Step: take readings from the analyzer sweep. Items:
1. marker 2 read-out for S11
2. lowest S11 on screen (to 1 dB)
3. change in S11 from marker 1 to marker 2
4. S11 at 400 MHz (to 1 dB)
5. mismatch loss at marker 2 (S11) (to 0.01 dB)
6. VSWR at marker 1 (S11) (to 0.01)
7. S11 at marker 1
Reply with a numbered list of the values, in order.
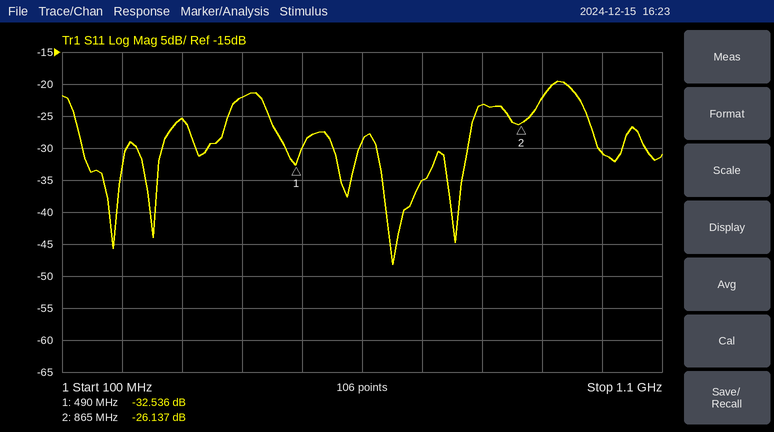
1. -26.137 dB
2. -48 dB
3. 6.399 dB
4. -22 dB
5. 0.01 dB
6. 1.05
7. -32.536 dB
